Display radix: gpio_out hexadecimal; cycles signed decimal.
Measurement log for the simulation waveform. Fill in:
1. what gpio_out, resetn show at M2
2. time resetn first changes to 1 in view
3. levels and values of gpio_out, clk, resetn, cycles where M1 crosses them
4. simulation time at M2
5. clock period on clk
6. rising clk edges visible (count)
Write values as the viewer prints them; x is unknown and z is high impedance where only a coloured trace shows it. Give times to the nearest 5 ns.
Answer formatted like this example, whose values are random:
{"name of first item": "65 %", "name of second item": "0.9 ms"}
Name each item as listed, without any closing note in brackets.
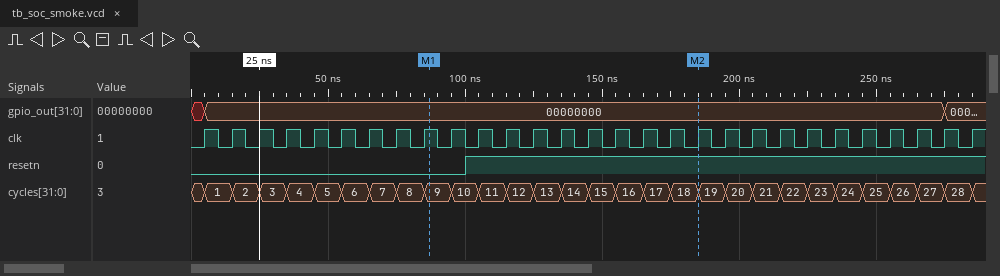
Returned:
{"what gpio_out, resetn show at M2": "gpio_out=00000000, resetn=1", "time resetn first changes to 1 in view": "100 ns", "levels and values of gpio_out, clk, resetn, cycles where M1 crosses them": "gpio_out=00000000, clk=1, resetn=0, cycles=9", "simulation time at M2": "185 ns", "clock period on clk": "10 ns", "rising clk edges visible": "29"}
